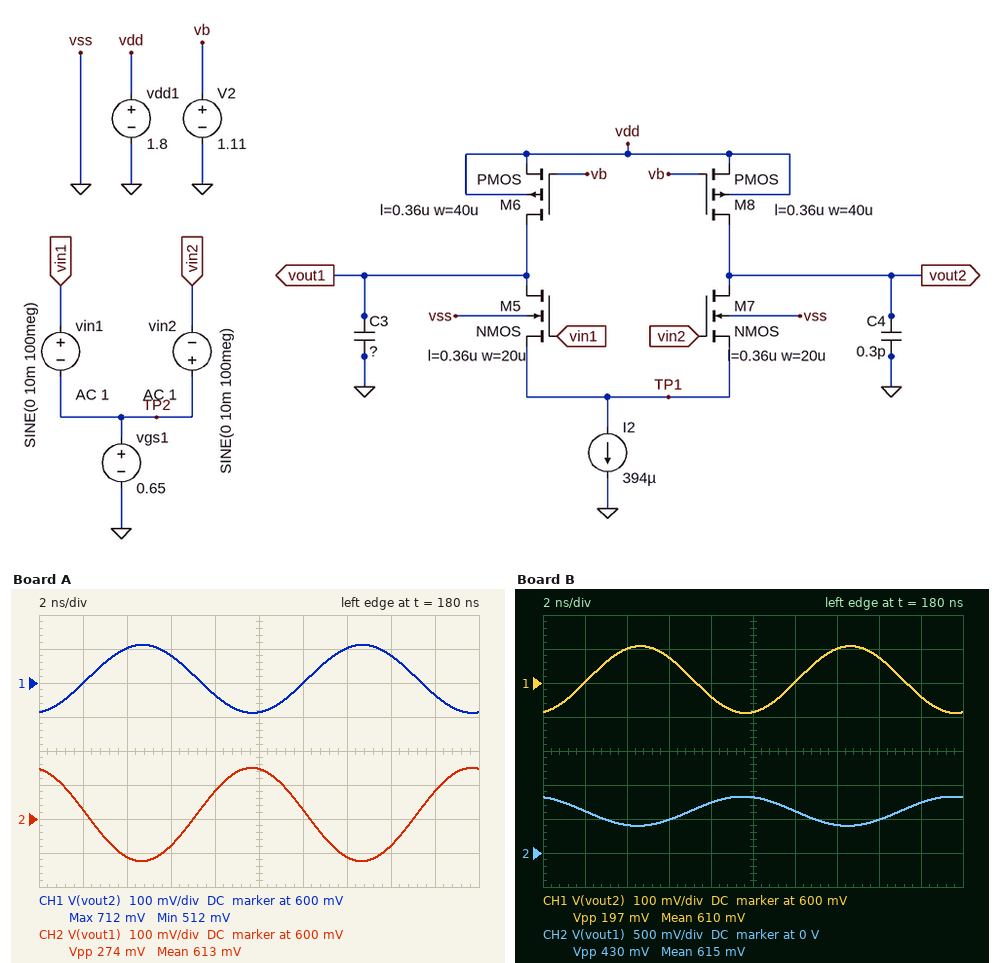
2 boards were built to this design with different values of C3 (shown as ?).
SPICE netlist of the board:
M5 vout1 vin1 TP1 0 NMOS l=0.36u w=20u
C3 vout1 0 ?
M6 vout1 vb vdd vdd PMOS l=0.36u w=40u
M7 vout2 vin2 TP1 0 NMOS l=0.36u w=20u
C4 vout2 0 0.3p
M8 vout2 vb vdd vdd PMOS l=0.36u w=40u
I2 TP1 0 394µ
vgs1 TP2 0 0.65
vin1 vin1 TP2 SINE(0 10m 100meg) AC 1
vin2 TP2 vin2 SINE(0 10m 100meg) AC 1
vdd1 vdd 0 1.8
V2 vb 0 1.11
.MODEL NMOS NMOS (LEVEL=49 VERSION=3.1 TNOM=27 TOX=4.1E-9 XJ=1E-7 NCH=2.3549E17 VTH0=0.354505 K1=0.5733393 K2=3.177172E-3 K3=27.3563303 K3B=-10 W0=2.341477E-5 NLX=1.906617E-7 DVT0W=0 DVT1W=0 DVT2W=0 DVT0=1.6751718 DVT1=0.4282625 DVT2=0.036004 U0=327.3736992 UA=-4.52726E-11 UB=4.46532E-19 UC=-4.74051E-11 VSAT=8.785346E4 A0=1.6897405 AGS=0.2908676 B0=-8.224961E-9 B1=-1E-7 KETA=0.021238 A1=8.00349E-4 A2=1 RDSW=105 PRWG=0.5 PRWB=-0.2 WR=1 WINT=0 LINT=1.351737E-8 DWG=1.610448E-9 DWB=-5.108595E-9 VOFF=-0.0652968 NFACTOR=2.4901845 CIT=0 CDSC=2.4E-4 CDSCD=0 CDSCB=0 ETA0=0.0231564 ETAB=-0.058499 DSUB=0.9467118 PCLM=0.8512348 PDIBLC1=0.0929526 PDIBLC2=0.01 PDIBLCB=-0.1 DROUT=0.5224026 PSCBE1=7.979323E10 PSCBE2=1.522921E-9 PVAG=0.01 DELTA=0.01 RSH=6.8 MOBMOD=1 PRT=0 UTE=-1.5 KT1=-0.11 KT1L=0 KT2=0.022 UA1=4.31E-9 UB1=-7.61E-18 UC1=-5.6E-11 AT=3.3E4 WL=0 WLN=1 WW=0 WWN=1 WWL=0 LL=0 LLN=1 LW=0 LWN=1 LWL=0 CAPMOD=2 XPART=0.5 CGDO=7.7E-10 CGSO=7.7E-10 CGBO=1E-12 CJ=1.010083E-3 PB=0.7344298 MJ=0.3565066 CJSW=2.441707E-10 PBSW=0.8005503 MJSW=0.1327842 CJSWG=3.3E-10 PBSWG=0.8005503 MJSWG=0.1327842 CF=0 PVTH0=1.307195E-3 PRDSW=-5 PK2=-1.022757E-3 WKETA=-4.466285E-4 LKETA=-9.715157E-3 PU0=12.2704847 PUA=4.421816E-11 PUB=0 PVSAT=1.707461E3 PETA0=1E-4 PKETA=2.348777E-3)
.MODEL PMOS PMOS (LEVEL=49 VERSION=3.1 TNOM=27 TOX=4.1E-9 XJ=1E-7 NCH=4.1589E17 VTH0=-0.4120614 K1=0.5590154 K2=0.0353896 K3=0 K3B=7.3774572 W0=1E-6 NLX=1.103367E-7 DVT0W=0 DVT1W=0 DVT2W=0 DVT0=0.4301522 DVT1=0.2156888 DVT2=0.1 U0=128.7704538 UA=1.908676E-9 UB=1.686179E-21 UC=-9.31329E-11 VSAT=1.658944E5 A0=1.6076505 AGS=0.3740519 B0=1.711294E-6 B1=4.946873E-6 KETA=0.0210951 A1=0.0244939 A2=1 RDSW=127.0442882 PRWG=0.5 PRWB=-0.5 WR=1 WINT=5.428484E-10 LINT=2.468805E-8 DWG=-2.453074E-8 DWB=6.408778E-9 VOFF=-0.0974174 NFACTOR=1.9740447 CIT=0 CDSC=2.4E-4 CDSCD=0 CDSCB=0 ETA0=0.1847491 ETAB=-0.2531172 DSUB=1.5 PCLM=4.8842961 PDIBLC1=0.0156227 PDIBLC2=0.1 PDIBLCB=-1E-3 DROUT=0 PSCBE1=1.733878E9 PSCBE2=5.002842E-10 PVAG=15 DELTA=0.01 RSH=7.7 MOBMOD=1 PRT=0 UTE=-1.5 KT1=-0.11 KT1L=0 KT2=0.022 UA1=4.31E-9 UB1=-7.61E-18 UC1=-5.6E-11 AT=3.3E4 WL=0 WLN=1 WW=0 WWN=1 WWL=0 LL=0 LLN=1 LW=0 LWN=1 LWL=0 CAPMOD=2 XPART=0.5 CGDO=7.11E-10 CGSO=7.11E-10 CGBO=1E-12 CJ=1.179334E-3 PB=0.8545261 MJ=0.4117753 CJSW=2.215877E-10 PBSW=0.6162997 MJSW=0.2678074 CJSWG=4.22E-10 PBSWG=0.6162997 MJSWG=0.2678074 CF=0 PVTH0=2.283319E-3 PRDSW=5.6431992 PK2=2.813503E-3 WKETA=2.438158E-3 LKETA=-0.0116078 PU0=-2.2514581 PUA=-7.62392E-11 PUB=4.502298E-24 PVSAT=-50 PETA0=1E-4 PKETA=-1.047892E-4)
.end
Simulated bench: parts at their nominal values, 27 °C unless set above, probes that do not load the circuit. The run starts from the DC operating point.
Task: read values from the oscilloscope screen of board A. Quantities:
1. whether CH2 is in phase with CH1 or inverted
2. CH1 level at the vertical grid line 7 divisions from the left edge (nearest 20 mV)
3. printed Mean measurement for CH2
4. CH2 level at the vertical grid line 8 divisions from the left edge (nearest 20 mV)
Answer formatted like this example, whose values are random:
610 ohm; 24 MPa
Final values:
inverted; 700 mV; 613 mV; 520 mV
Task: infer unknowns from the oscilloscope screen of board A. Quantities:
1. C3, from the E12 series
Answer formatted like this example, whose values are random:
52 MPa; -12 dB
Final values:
220 fF
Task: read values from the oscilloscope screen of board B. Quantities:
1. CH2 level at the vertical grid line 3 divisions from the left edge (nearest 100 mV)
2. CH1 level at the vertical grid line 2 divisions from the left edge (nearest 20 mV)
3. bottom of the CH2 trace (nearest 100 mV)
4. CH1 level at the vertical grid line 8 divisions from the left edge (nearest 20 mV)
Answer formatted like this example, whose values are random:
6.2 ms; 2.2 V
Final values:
500 mV; 700 mV; 400 mV; 680 mV
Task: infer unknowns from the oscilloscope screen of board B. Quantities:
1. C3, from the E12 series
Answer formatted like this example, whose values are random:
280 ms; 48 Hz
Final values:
120 fF
